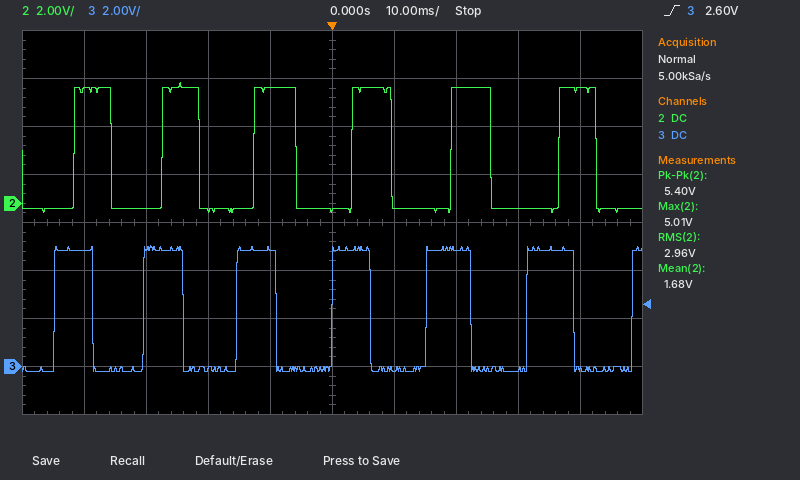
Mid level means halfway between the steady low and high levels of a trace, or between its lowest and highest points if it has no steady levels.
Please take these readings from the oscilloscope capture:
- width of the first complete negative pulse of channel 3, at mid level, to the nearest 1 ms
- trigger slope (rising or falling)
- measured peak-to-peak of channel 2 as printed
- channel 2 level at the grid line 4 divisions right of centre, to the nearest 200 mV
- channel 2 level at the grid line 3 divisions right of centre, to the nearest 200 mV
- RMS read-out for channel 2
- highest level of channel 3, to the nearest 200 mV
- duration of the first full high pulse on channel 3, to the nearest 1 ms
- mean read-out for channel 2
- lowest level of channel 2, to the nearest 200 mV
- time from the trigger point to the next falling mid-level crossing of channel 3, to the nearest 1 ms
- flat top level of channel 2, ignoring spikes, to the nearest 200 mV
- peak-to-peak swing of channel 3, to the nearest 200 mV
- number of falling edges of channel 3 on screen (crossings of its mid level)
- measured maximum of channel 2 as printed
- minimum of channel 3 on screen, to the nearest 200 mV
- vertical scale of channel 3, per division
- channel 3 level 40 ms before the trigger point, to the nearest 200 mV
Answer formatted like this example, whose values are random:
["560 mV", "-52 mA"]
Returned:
["8 ms", "rising", "5.40 V", "4.8 V", "-200 mV", "2.96 V", "5.0 V", "6 ms", "1.68 V", "-400 mV", "6 ms", "4.8 V", "5.2 V", "6", "5.01 V", "-200 mV", "2 V", "4.8 V"]
